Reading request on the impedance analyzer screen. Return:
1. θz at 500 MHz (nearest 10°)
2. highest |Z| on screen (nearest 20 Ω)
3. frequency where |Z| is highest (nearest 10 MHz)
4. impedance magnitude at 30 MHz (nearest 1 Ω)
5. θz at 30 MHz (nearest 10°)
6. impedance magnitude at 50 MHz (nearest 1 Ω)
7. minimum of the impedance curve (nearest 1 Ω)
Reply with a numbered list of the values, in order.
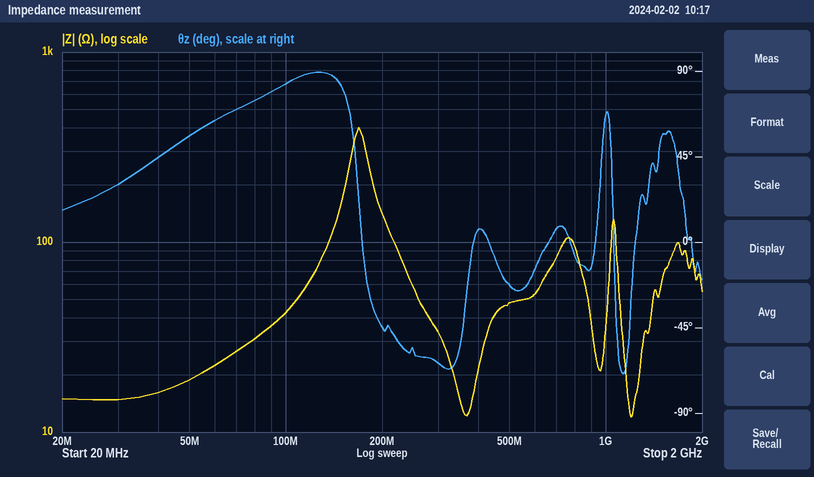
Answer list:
1. -20°
2. 400 Ω
3. 170 MHz
4. 15 Ω
5. 30°
6. 19 Ω
7. 12 Ω
